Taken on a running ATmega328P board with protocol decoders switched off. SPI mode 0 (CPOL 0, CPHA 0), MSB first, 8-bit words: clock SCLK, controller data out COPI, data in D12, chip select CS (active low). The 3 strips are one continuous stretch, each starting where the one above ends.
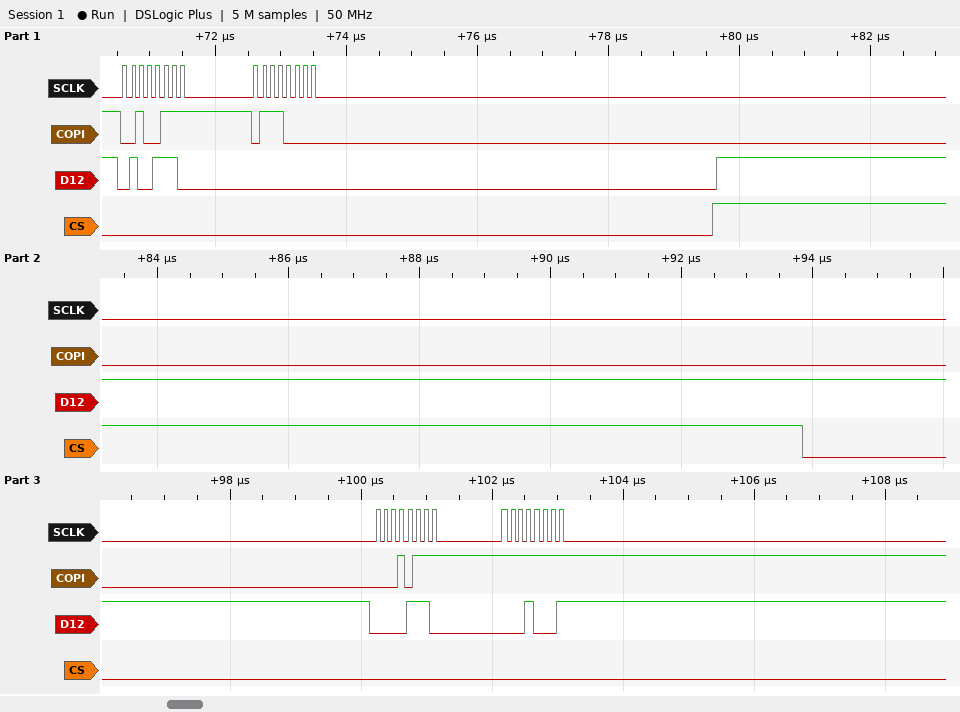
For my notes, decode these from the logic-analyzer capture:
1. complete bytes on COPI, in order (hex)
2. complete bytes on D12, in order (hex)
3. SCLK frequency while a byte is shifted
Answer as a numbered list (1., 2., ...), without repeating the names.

1. 0x27 0x70 0x17 0xFF
2. 0x4E 0x00 0x0E 0x11
3. 8 MHz
